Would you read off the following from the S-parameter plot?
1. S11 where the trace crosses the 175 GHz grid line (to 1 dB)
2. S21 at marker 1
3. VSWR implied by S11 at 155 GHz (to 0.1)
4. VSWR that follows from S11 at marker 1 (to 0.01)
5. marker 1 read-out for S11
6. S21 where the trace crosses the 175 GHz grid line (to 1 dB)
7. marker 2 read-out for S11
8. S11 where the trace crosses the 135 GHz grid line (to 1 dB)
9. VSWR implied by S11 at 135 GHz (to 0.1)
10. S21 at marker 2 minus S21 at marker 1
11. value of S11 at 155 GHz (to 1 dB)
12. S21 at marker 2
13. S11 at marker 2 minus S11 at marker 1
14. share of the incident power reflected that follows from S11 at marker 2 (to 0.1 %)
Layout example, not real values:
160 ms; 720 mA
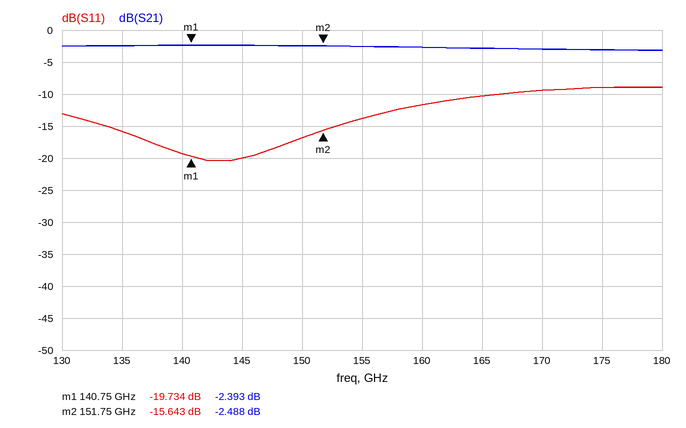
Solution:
-9 dB; -2.393 dB; 1.5; 1.23; -19.734 dB; -3 dB; -15.643 dB; -16 dB; 1.4; -0.095 dB; -14 dB; -2.488 dB; 4.091 dB; 2.7 %
